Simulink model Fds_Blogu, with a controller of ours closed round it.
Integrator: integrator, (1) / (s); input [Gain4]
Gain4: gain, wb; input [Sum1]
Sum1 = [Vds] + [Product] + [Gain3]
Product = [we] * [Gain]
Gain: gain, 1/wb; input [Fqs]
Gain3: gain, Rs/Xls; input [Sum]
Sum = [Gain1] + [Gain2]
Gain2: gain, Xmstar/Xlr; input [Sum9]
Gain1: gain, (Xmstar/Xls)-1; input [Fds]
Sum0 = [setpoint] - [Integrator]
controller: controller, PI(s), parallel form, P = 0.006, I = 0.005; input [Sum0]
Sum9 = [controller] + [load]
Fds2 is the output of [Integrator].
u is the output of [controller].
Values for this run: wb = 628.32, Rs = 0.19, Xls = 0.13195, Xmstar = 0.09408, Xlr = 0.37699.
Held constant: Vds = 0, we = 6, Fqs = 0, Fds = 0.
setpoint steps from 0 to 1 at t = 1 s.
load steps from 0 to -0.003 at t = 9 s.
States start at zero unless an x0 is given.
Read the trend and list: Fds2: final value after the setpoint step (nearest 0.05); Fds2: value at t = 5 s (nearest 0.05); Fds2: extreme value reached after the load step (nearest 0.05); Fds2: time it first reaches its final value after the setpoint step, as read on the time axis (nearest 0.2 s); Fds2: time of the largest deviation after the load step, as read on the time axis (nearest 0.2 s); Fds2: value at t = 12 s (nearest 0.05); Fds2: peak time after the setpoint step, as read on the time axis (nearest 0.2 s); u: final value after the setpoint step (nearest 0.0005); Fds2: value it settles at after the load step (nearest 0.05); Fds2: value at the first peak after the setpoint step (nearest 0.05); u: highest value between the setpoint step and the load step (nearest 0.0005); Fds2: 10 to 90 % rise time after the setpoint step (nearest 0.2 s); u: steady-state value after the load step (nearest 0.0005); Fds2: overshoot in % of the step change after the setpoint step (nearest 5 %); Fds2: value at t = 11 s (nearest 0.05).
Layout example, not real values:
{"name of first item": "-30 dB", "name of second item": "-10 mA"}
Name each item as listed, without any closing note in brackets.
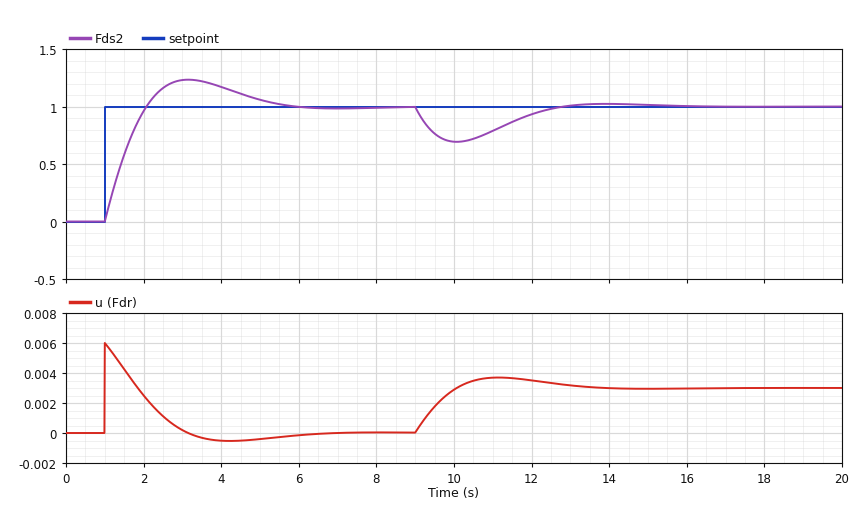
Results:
{"Fds2: final value after the setpoint step": "1.00", "Fds2: value at t = 5 s": "1.05", "Fds2: extreme value reached after the load step": "0.70", "Fds2: time it first reaches its final value after the setpoint step, as read on the time axis": "2.0 s", "Fds2: time of the largest deviation after the load step, as read on the time axis": "10.0 s", "Fds2: value at t = 12 s": "0.95", "Fds2: peak time after the setpoint step, as read on the time axis": "3.2 s", "u: final value after the setpoint step": "0.0000", "Fds2: value it settles at after the load step": "1.00", "Fds2: value at the first peak after the setpoint step": "1.25", "u: highest value between the setpoint step and the load step": "0.0060", "Fds2: 10 to 90 % rise time after the setpoint step": "0.8 s", "u: steady-state value after the load step": "0.0030", "Fds2: overshoot in % of the step change after the setpoint step": "25 %", "Fds2: value at t = 11 s": "0.80"}
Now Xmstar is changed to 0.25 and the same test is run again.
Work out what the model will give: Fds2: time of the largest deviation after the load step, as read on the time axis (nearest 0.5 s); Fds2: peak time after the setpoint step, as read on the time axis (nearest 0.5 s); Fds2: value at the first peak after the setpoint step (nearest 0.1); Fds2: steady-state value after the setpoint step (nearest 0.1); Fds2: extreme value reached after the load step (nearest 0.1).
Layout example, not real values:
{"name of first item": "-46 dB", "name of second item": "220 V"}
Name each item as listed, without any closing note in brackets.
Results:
{"Fds2: time of the largest deviation after the load step, as read on the time axis": "9.5 s", "Fds2: peak time after the setpoint step, as read on the time axis": "2.0 s", "Fds2: value at the first peak after the setpoint step": "1.1", "Fds2: steady-state value after the setpoint step": "1.0", "Fds2: extreme value reached after the load step": "0.6"}
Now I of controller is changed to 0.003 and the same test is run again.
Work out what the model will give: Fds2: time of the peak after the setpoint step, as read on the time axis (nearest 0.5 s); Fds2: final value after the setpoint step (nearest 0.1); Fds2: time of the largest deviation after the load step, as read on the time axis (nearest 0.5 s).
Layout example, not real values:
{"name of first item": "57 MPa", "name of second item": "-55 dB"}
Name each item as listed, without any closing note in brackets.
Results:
{"Fds2: time of the peak after the setpoint step, as read on the time axis": "3.5 s", "Fds2: final value after the setpoint step": "1.0", "Fds2: time of the largest deviation after the load step, as read on the time axis": "10.5 s"}
